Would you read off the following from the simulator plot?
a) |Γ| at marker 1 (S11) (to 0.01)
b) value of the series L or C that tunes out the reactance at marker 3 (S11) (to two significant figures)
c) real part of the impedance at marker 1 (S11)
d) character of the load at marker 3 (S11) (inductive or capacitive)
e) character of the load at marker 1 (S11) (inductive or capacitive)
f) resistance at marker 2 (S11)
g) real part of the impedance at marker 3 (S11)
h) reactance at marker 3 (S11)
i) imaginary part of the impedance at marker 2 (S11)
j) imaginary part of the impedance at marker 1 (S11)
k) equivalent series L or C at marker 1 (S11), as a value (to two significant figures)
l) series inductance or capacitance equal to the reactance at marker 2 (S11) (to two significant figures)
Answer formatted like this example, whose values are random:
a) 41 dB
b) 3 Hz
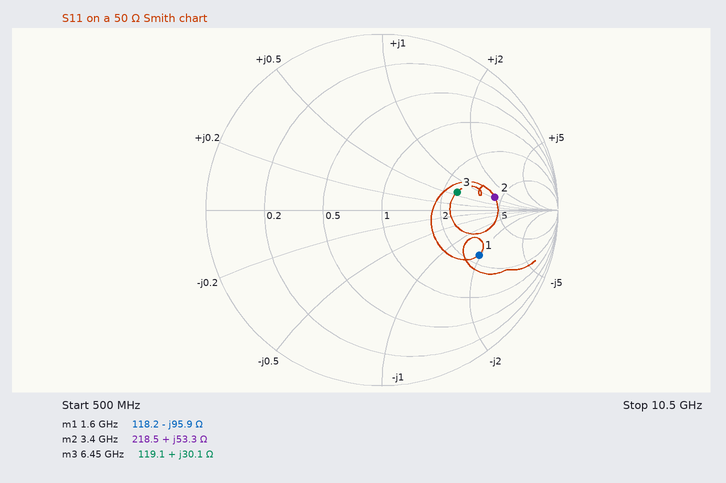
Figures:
a) 0.61
b) 820 fF
c) 118.2 Ω
d) inductive
e) capacitive
f) 218.5 Ω
g) 119.1 Ω
h) +30.1 Ω
i) +53.3 Ω
j) -95.9 Ω
k) 1.0 pF
l) 2.5 nH
